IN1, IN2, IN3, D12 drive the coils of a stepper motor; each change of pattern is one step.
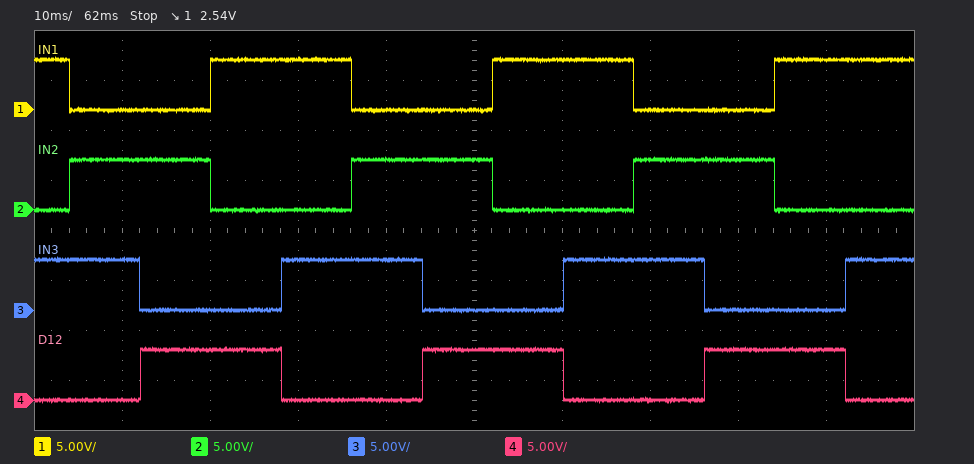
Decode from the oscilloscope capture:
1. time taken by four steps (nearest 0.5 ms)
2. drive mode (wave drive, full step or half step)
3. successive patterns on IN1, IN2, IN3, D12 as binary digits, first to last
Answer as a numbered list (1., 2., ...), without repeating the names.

1. 32.0 ms
2. full step
3. 1010 0110 0101 1001 1010 0110 0101 1001 1010 0110 0101 1001 1010
